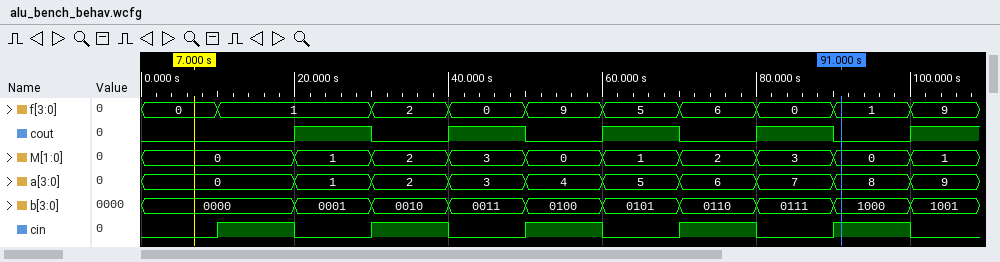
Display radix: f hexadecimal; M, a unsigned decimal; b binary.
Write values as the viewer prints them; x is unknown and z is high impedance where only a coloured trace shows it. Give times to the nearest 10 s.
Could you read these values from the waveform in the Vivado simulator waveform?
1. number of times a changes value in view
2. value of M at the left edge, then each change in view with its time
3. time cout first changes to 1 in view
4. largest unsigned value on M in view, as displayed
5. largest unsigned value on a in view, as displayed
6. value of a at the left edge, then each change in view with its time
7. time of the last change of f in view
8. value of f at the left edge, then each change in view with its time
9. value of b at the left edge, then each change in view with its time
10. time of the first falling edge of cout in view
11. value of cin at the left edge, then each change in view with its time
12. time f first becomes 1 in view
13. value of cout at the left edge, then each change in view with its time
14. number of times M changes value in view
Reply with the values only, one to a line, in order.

9
0, 1 at 20 s, 2 at 30 s, 3 at 40 s, 0 at 50 s, 1 at 60 s, 2 at 70 s, 3 at 80 s, 0 at 90 s, 1 at 100 s
20 s
3
9
0, 1 at 20 s, 2 at 30 s, 3 at 40 s, 4 at 50 s, 5 at 60 s, 6 at 70 s, 7 at 80 s, 8 at 90 s, 9 at 100 s
100 s
0, 1 at 10 s, 2 at 30 s, 0 at 40 s, 9 at 50 s, 5 at 60 s, 6 at 70 s, 0 at 80 s, 1 at 90 s, 9 at 100 s
0000, 0001 at 20 s, 0010 at 30 s, 0011 at 40 s, 0100 at 50 s, 0101 at 60 s, 0110 at 70 s, 0111 at 80 s, 1000 at 90 s, 1001 at 100 s
30 s
0, 1 at 10 s, 0 at 20 s, 1 at 30 s, 0 at 40 s, 1 at 50 s, 0 at 60 s, 1 at 70 s, 0 at 80 s, 1 at 90 s, 0 at 100 s
10 s
0, 1 at 20 s, 0 at 30 s, 1 at 40 s, 0 at 50 s, 1 at 60 s, 0 at 70 s, 1 at 80 s, 0 at 90 s, 1 at 100 s
9
